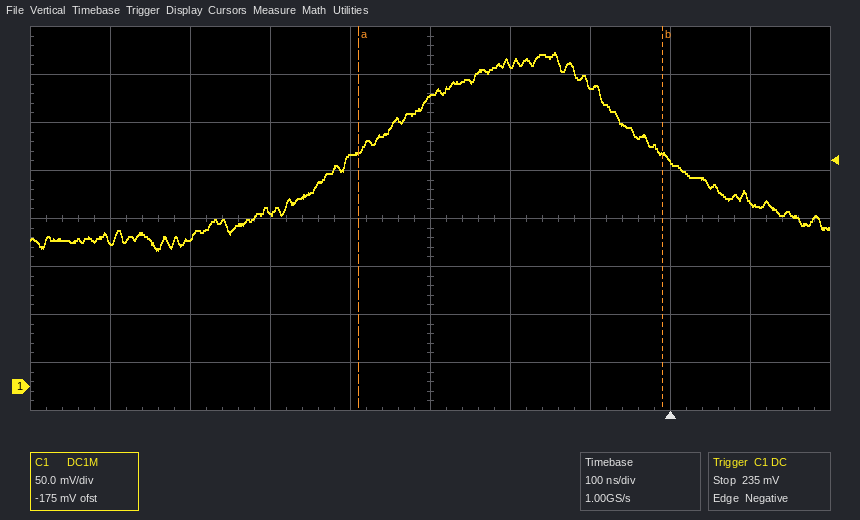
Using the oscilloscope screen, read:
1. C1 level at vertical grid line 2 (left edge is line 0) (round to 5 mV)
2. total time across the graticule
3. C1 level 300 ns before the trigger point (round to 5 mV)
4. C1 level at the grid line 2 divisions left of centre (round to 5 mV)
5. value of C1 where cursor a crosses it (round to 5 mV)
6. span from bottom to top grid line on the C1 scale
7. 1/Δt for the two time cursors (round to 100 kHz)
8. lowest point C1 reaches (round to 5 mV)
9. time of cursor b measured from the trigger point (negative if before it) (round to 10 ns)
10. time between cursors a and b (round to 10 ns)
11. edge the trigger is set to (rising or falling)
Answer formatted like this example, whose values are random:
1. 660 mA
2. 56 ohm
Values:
1. 155 mV
2. 1 µs
3. 300 mV
4. 180 mV
5. 245 mV
6. 400 mV
7. 2.6 MHz
8. 140 mV
9. -10 ns
10. 380 ns
11. falling
